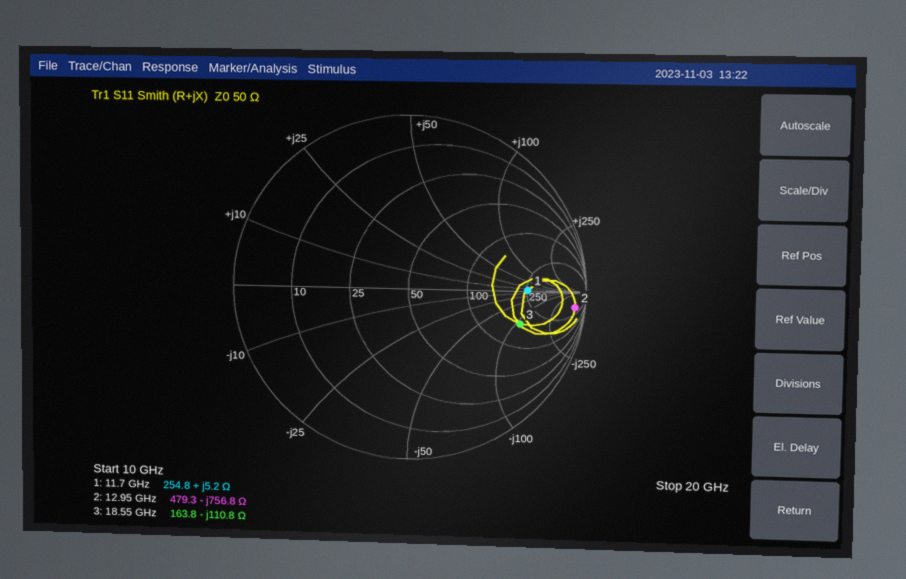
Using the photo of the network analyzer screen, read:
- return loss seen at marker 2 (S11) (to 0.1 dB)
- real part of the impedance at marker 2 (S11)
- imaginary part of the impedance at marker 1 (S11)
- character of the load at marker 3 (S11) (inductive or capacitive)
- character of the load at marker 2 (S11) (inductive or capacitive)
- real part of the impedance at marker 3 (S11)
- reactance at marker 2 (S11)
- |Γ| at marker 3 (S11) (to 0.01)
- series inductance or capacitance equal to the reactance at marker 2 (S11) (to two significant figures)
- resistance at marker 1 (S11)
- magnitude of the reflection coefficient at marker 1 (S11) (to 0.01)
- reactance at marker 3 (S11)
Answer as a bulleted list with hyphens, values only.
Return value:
- 0.5 dB
- 479.3 Ω
- +5.2 Ω
- capacitive
- capacitive
- 163.8 Ω
- -756.8 Ω
- 0.66
- 16 fF
- 254.8 Ω
- 0.67
- -110.8 Ω
